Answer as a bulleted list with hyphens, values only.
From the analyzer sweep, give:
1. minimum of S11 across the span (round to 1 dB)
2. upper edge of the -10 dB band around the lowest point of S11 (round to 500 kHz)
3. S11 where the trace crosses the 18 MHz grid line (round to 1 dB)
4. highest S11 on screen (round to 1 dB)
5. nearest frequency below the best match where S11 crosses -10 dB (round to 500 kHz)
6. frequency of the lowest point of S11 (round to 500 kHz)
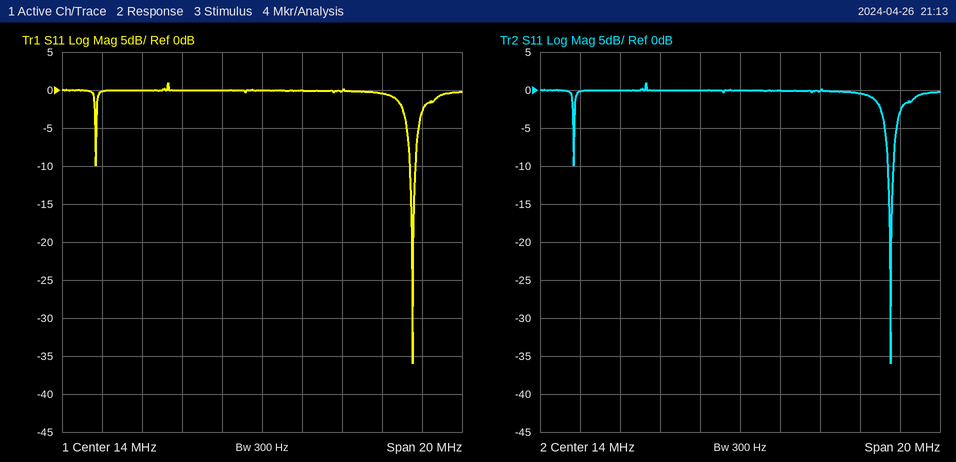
- -36 dB
- 21.5 MHz
- 0 dB
- 1 dB
- 21.5 MHz
- 21.5 MHz
